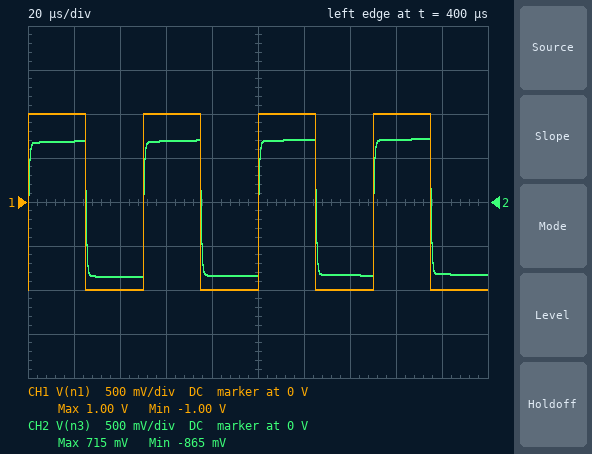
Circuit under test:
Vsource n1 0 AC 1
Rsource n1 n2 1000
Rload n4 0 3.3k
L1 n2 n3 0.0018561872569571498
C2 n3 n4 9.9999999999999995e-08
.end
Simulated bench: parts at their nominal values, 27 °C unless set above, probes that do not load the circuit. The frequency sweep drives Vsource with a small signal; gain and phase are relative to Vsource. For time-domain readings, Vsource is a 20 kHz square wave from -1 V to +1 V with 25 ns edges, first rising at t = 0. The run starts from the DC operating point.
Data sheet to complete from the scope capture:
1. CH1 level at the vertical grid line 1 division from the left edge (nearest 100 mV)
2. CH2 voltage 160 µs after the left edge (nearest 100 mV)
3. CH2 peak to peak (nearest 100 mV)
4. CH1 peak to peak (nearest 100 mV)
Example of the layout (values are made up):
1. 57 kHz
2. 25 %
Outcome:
1. 1.0 V
2. 700 mV
3. 1.6 V
4. 2.0 V
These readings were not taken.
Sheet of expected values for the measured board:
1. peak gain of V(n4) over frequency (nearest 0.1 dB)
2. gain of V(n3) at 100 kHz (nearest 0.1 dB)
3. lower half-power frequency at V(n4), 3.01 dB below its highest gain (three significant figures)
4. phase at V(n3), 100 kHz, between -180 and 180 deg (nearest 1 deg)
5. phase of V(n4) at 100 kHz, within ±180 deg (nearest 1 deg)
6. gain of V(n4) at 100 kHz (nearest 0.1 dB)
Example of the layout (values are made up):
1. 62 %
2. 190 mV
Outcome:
1. -2.3 dB
2. -2.6 dB
3. 370 Hz
4. -15 deg
5. -15 deg
6. -2.6 dB
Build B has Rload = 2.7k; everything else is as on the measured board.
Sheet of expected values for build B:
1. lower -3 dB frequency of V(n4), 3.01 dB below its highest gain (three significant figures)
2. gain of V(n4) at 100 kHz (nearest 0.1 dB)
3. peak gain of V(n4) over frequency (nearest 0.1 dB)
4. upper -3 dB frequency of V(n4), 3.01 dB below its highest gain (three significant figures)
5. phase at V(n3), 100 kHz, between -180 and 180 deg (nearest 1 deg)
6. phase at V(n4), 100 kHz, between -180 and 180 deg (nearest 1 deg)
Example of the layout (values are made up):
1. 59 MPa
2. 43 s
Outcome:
1. 430 Hz
2. -3.1 dB
3. -2.7 dB
4. 318 kHz
5. -18 deg
6. -17 deg
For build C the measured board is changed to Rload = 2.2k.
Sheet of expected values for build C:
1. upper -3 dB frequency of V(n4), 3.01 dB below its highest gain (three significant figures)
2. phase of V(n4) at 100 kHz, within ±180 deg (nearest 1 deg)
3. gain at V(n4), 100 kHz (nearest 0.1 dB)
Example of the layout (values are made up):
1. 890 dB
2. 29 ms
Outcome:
1. 275 kHz
2. -20 deg
3. -3.8 dB
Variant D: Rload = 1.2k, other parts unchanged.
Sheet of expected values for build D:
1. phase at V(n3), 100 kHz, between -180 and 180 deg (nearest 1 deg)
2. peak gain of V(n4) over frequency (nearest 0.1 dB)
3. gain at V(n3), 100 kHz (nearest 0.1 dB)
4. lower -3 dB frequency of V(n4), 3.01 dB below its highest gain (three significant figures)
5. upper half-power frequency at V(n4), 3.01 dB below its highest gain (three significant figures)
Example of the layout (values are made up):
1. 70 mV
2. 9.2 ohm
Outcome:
1. -28 deg
2. -5.3 dB
3. -6.3 dB
4. 721 Hz
5. 189 kHz
